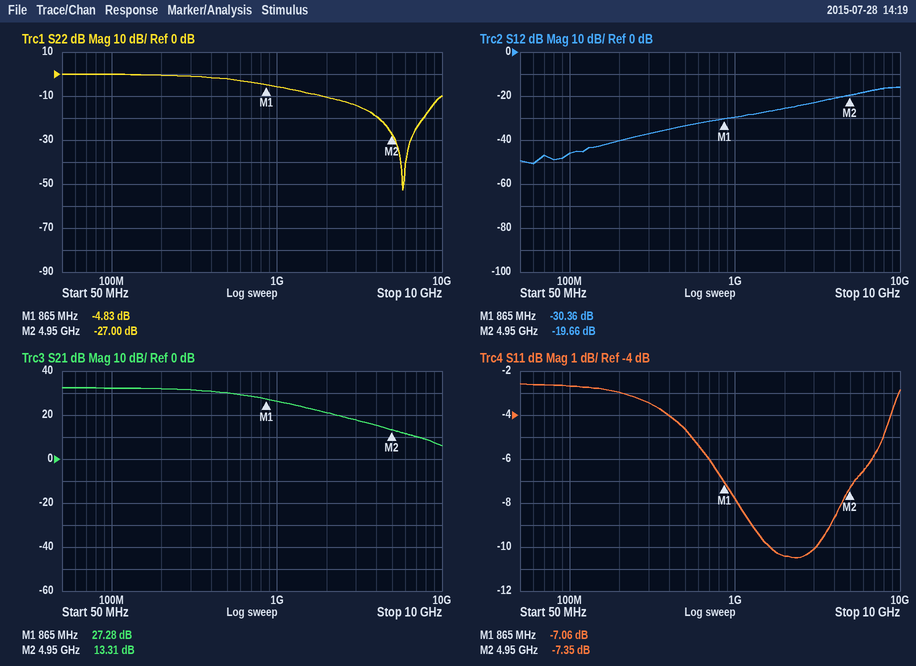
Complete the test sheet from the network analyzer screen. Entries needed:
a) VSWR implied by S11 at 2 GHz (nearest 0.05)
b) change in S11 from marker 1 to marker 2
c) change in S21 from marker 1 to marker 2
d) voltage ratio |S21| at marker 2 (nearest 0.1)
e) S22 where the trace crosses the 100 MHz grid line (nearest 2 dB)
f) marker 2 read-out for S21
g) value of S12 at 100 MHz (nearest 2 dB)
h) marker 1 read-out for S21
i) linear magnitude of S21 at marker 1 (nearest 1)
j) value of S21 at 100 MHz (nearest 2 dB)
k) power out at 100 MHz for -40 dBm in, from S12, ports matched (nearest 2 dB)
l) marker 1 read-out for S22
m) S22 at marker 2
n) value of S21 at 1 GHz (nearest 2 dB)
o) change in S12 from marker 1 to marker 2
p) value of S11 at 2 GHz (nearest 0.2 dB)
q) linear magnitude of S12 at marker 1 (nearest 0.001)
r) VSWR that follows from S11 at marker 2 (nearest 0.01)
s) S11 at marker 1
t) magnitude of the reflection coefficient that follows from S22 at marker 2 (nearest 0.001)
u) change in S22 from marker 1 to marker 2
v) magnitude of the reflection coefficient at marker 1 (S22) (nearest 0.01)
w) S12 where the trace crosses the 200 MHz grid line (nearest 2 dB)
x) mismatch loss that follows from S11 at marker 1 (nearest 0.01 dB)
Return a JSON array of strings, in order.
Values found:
["1.85", "-0.29 dB", "-13.97 dB", "4.6", "0 dB", "13.31 dB", "-46 dB", "27.28 dB", "23", "32 dB", "-86 dBm", "-4.83 dB", "-27.00 dB", "26 dB", "10.70 dB", "-10.4 dB", "0.030", "2.50", "-7.06 dB", "0.045", "-22.17 dB", "0.57", "-40 dB", "0.95 dB"]
